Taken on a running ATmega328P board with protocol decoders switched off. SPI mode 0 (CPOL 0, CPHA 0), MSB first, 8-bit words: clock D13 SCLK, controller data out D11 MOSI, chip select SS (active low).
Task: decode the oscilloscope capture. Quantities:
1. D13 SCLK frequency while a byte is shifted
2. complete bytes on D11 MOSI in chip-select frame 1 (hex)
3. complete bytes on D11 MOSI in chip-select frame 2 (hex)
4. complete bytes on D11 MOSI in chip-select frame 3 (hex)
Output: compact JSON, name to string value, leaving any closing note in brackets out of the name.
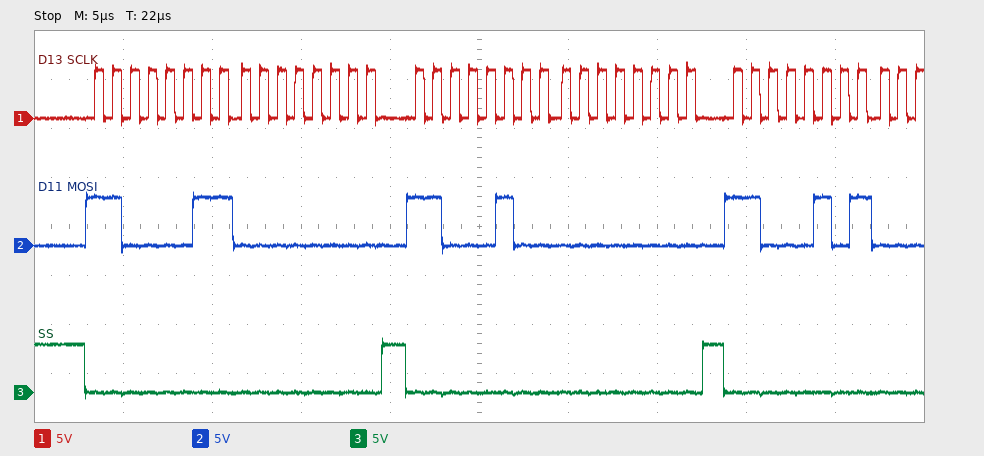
{"D13 SCLK frequency while a byte is shifted": "1 MHz", "complete bytes on D11 MOSI in chip-select frame 1": "C3 00", "complete bytes on D11 MOSI in chip-select frame 2": "C4 00", "complete bytes on D11 MOSI in chip-select frame 3": "C5"}
